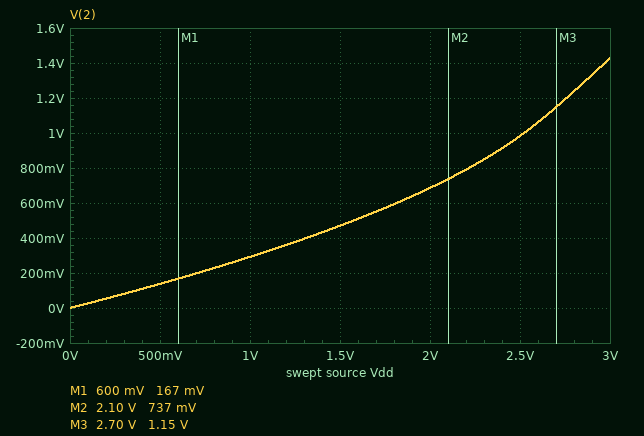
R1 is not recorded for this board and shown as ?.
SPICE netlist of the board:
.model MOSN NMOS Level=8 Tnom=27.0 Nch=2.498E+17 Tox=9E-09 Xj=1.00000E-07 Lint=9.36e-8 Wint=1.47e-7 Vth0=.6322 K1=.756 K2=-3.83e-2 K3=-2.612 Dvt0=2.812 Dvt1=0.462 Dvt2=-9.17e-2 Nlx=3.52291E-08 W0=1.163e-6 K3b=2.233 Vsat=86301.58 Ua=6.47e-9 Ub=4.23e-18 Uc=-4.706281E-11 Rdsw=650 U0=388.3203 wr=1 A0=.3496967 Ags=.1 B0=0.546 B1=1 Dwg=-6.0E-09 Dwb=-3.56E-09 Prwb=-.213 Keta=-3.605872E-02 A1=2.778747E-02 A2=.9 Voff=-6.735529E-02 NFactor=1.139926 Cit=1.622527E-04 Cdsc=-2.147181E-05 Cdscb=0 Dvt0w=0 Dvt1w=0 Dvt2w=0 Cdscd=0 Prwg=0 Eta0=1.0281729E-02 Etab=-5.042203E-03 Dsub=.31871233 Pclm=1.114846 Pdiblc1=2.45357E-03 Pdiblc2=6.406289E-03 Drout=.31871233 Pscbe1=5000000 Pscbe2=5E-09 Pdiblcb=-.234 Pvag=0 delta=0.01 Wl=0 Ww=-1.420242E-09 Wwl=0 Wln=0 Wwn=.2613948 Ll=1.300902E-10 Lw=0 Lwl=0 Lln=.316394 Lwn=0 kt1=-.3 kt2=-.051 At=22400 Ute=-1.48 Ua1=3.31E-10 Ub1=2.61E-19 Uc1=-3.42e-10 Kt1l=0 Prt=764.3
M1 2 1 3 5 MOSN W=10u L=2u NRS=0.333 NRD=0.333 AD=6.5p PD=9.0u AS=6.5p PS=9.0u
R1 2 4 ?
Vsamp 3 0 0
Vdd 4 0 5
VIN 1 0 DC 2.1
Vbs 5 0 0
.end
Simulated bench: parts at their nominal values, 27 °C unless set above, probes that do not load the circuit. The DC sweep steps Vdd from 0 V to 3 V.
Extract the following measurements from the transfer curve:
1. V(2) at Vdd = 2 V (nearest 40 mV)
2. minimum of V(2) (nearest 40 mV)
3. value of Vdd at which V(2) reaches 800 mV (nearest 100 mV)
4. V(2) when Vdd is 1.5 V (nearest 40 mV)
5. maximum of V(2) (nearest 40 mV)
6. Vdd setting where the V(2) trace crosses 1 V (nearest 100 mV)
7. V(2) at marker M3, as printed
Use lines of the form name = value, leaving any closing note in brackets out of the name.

V(2) at Vdd = 2 V = 680 mV
minimum of V(2) = 0 V
value of Vdd at which V(2) reaches 800 mV = 2.2 V
V(2) when Vdd is 1.5 V = 480 mV
maximum of V(2) = 1.44 V
Vdd setting where the V(2) trace crosses 1 V = 2.5 V
V(2) at marker M3, as printed = 1.15 V
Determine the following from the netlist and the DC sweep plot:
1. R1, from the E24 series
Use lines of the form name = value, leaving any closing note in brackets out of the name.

R1, from the E24 series = 8.2 kΩ
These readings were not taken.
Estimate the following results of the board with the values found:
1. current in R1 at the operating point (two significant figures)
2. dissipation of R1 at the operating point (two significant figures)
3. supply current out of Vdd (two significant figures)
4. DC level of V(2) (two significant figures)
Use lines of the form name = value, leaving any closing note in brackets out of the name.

current in R1 at the operating point = 200 µA
dissipation of R1 at the operating point = 320 µW
supply current out of Vdd = 200 µA
DC level of V(2) = 3.4 V
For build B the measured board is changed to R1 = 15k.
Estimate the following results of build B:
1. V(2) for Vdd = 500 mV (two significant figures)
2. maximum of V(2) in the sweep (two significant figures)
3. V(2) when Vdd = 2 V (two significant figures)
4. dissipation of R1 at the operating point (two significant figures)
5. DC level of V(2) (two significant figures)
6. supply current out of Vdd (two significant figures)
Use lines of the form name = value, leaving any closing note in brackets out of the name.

V(2) for Vdd = 500 mV = 84 mV
maximum of V(2) in the sweep = 660 mV
V(2) when Vdd = 2 V = 380 mV
dissipation of R1 at the operating point = 570 µW
DC level of V(2) = 2.1 V
supply current out of Vdd = 190 µA
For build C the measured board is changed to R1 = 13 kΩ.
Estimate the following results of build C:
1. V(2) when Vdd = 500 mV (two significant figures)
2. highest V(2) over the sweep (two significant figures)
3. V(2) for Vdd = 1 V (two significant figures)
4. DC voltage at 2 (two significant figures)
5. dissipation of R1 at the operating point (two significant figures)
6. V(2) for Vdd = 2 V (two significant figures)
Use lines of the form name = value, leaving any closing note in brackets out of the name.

V(2) when Vdd = 500 mV = 95 mV
highest V(2) over the sweep = 780 mV
V(2) for Vdd = 1 V = 200 mV
DC voltage at 2 = 2.5 V
dissipation of R1 at the operating point = 500 µW
V(2) for Vdd = 2 V = 440 mV
